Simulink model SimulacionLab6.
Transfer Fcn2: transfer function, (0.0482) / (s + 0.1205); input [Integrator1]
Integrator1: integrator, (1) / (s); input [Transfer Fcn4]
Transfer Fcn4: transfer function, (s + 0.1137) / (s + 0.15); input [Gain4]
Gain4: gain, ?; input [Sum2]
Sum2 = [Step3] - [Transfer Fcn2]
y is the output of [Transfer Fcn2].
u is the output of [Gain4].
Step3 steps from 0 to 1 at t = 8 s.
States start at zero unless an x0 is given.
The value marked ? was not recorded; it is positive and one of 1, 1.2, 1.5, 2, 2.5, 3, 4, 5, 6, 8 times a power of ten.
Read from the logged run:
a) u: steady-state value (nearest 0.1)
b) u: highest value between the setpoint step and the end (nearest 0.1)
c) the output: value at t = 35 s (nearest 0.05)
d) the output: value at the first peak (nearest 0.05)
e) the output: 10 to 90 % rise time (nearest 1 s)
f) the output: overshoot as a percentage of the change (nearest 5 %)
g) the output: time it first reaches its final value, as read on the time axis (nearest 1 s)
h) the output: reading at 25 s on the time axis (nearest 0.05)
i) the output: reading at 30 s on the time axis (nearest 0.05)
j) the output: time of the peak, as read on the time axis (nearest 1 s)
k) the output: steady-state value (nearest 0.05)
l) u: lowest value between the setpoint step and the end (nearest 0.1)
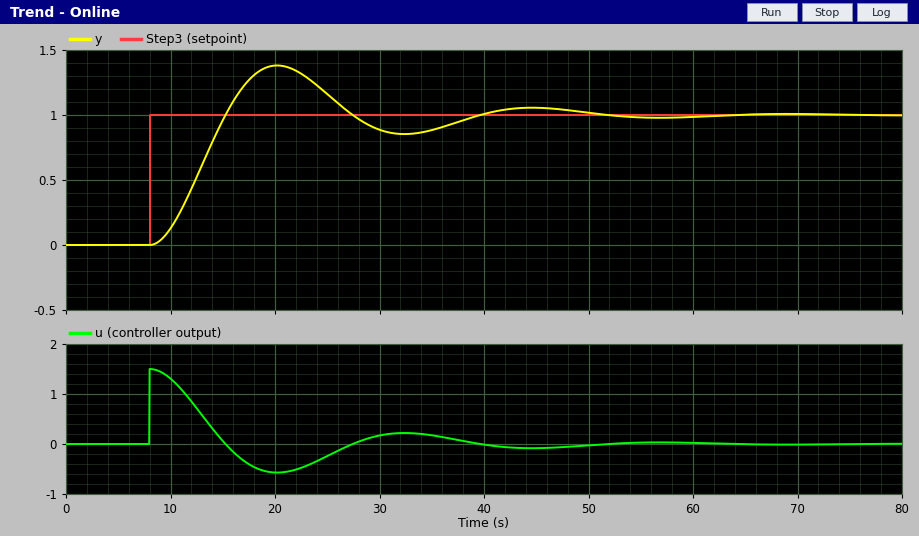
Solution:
0.0
1.5
0.90
1.40
5 s
40 %
15 s
1.15
0.90
20 s
1.00
-0.6
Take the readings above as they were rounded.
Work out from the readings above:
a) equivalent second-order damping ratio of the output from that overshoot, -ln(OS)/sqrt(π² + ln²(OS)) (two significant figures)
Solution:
0.28
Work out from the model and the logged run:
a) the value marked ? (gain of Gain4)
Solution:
1.5
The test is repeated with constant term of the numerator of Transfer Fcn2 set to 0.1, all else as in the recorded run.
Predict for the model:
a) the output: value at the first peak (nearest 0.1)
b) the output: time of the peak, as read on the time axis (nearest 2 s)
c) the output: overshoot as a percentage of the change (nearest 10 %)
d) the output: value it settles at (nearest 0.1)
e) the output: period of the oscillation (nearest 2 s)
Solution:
1.5
16 s
50 %
1.0
16 s
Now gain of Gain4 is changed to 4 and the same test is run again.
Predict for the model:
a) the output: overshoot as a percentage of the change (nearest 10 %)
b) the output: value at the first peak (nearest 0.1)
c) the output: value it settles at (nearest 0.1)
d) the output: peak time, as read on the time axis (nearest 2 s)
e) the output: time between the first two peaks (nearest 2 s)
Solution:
60 %
1.6
1.0
16 s
14 s
